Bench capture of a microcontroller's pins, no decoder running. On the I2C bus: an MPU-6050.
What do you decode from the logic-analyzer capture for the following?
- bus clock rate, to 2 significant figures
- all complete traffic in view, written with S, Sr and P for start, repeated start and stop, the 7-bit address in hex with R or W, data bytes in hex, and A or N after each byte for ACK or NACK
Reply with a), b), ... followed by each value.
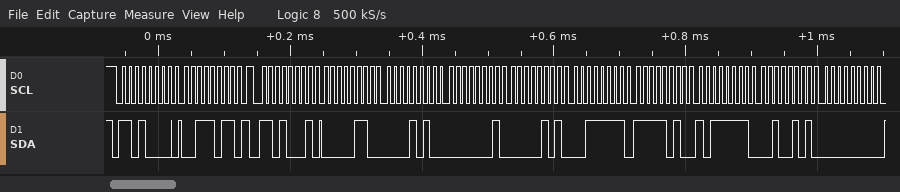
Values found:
a) 100 kHz
b) S 68W A 3B A Sr 68R A 06 A 0A A 01 A 05 A 3F A FA A BF A 25 A 00 A
